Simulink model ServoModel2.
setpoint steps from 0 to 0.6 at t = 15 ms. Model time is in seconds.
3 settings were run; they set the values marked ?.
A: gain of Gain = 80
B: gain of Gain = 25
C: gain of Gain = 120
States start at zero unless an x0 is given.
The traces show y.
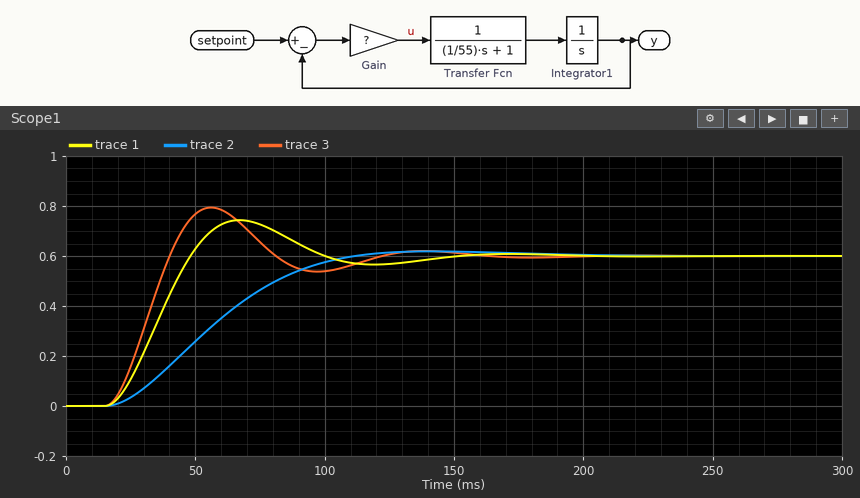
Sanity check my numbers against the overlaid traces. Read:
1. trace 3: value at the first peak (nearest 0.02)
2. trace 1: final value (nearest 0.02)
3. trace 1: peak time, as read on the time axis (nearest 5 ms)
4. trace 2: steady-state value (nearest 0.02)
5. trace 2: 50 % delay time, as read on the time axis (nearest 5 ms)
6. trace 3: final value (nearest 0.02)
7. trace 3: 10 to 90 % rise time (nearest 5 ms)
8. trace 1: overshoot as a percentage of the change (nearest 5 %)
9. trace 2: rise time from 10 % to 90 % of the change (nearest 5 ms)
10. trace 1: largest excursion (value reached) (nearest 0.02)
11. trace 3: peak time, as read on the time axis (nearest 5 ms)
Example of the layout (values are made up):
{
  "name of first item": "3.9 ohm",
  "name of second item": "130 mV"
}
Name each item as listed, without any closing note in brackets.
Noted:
{
  "trace 3: value at the first peak": "0.80",
  "trace 1: final value": "0.60",
  "trace 1: peak time, as read on the time axis": "65 ms",
  "trace 2: steady-state value": "0.60",
  "trace 2: 50 % delay time, as read on the time axis": "55 ms",
  "trace 3: final value": "0.60",
  "trace 3: 10 to 90 % rise time": "15 ms",
  "trace 1: overshoot as a percentage of the change": "25 %",
  "trace 2: rise time from 10 % to 90 % of the change": "60 ms",
  "trace 1: largest excursion (value reached)": "0.74",
  "trace 3: peak time, as read on the time axis": "55 ms"
}
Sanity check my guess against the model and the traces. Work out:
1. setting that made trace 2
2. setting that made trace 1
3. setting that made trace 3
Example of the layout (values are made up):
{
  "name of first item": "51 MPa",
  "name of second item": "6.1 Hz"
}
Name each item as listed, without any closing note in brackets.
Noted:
{
  "setting that made trace 2": "B",
  "setting that made trace 1": "A",
  "setting that made trace 3": "C"
}
